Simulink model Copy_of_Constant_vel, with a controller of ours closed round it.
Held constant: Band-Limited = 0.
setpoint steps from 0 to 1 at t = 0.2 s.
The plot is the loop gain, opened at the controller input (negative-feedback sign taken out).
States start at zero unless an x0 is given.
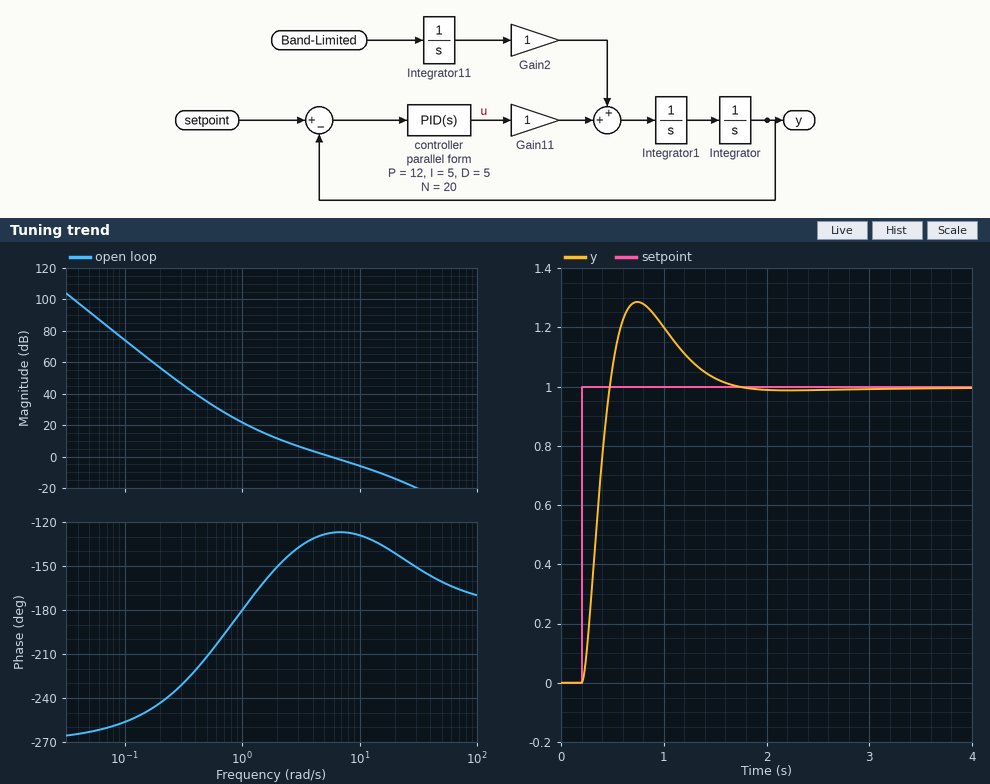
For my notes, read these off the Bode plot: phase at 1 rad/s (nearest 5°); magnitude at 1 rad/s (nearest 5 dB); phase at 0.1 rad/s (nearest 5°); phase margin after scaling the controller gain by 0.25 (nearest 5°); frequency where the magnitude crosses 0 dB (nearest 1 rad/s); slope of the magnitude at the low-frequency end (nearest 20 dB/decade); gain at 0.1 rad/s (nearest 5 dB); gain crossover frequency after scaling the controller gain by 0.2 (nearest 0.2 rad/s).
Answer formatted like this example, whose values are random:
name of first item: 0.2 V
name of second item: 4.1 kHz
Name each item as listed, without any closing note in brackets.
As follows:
phase at 1 rad/s: -180°
magnitude at 1 rad/s: 20 dB
phase at 0.1 rad/s: -255°
phase margin after scaling the controller gain by 0.25: 30°
frequency where the magnitude crosses 0 dB: 6 rad/s
slope of the magnitude at the low-frequency end: -60 dB/decade
gain at 0.1 rad/s: 75 dB
gain crossover frequency after scaling the controller gain by 0.2: 1.6 rad/s
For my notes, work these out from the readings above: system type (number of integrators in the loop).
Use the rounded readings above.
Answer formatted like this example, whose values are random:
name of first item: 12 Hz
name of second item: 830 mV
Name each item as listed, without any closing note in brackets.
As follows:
system type: 3
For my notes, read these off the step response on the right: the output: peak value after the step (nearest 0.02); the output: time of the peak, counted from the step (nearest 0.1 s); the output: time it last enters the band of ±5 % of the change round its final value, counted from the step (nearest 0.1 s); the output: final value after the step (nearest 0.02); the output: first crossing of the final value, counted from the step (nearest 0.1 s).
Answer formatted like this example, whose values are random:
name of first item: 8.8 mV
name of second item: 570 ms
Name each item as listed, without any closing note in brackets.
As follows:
the output: peak value after the step: 1.28
the output: time of the peak, counted from the step: 0.5 s
the output: time it last enters the band of ±5 % of the change round its final value, counted from the step: 1.2 s
the output: final value after the step: 1.00
the output: first crossing of the final value, counted from the step: 0.3 s
